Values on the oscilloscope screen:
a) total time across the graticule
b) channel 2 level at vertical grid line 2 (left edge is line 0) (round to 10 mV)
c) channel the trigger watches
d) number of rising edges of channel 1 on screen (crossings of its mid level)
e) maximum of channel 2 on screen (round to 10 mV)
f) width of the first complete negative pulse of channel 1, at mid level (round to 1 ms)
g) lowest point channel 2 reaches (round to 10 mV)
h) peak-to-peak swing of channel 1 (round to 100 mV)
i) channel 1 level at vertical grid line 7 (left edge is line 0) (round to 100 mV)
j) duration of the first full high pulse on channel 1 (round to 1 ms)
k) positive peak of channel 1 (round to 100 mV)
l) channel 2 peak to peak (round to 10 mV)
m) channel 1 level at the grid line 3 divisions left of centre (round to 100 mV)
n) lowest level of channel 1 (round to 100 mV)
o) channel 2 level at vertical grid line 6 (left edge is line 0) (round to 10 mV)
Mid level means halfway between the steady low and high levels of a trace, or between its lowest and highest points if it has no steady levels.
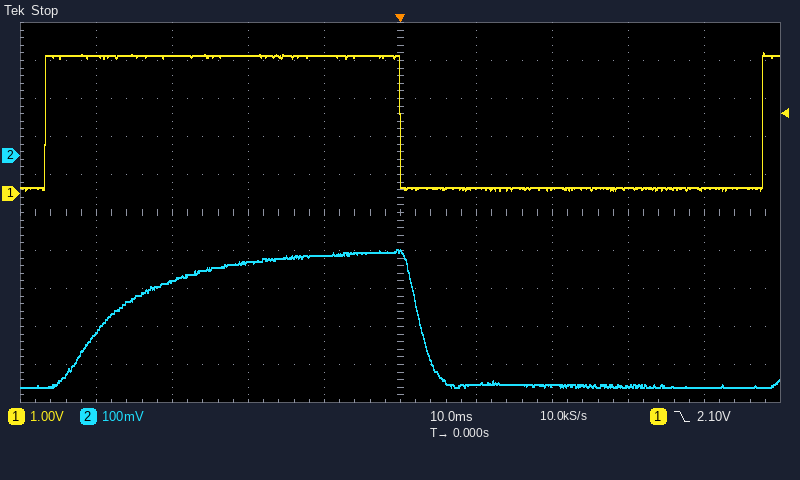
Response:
100 ms
-330 mV
channel 1
2
-250 mV
48 ms
-610 mV
3.6 V
100 mV
47 ms
3.7 V
360 mV
3.6 V
100 mV
-600 mV
